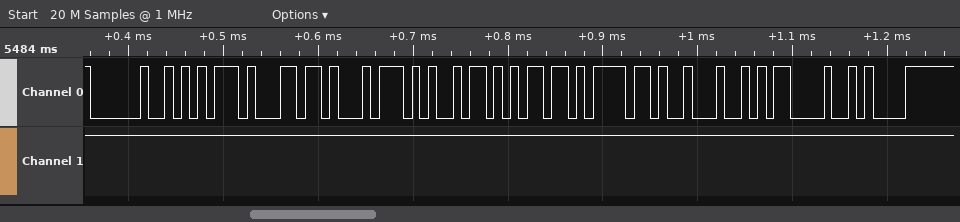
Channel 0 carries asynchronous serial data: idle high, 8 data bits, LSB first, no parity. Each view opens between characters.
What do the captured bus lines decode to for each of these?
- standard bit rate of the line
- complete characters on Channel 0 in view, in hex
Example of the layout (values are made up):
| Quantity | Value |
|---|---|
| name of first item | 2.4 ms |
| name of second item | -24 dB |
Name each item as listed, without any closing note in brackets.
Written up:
| Quantity | Value |
|---|---|
| standard bit rate of the line | 115200 baud |
| complete characters on Channel 0 in view, in hex | 20, 75, 6C, 74, 69, 6D, 6F, 22, 0D, 0A |
